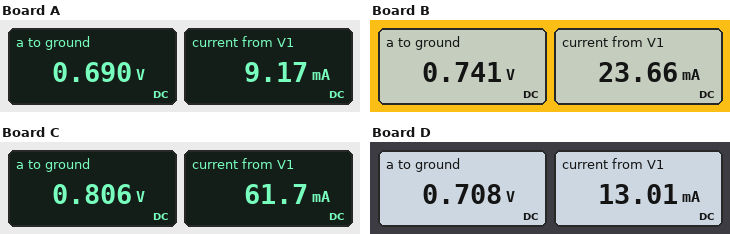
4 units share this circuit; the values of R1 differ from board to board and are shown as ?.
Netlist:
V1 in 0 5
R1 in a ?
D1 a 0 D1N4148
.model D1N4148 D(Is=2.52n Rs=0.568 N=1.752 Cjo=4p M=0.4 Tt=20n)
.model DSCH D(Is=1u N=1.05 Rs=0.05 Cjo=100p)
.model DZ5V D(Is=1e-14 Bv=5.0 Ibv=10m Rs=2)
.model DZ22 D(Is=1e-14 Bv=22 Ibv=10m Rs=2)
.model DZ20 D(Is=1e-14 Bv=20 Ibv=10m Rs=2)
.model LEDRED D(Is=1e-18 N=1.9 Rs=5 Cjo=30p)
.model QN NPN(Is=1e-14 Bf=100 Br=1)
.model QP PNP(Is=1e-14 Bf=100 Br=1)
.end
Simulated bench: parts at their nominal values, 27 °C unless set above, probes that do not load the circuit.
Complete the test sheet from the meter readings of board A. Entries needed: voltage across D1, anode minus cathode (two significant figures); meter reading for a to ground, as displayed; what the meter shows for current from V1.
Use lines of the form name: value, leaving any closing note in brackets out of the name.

voltage across D1, anode minus cathode: 690 mV
meter reading for a to ground, as displayed: 0.690 V
what the meter shows for current from V1: 9.17 mA
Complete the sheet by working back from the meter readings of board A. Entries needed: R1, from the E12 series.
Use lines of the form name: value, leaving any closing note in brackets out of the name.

R1, from the E12 series: 470 Ω
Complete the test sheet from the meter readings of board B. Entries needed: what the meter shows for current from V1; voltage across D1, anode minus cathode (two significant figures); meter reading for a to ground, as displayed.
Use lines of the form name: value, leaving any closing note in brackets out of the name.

what the meter shows for current from V1: 23.66 mA
voltage across D1, anode minus cathode: 740 mV
meter reading for a to ground, as displayed: 0.741 V
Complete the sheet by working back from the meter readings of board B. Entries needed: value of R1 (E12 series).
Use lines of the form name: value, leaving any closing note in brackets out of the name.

value of R1: 180 Ω
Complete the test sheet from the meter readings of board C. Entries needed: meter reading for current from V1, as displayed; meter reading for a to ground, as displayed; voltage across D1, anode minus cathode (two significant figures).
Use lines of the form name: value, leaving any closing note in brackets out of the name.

meter reading for current from V1, as displayed: 61.7 mA
meter reading for a to ground, as displayed: 0.806 V
voltage across D1, anode minus cathode: 810 mV
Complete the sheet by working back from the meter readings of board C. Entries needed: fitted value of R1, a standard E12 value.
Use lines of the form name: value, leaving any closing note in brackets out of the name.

fitted value of R1, a standard E12 value: 68 Ω
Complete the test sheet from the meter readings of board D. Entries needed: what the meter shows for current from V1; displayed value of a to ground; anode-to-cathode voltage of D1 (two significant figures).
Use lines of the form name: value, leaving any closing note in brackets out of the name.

what the meter shows for current from V1: 13.01 mA
displayed value of a to ground: 0.708 V
anode-to-cathode voltage of D1: 710 mV
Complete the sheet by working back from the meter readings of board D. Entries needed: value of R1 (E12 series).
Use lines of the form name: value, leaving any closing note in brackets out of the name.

value of R1: 330 Ω
